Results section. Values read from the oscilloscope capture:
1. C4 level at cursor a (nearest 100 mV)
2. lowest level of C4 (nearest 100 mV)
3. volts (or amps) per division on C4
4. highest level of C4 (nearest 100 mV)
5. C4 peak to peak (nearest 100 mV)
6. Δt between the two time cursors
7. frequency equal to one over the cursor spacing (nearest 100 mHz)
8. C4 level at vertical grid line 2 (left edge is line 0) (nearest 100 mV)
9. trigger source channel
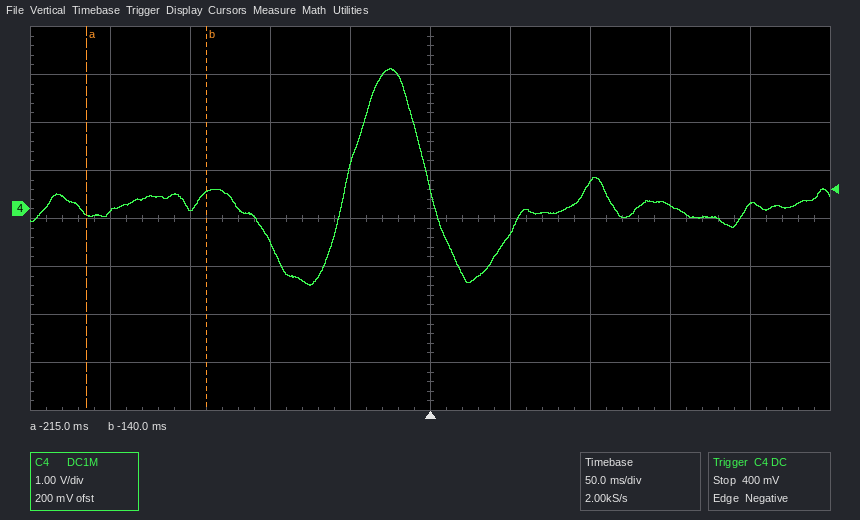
-100 mV
-1.6 V
1 V
2.9 V
4.5 V
75 ms
13.3 Hz
0.0 V
C4
